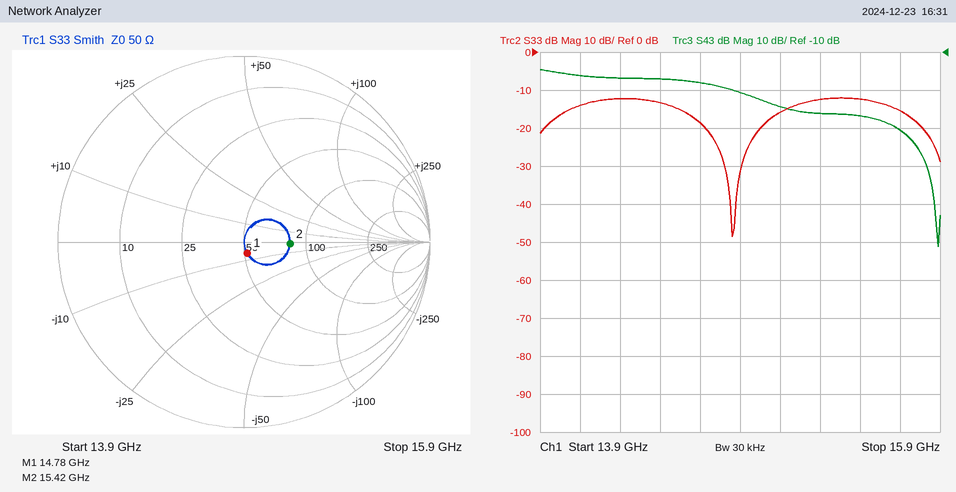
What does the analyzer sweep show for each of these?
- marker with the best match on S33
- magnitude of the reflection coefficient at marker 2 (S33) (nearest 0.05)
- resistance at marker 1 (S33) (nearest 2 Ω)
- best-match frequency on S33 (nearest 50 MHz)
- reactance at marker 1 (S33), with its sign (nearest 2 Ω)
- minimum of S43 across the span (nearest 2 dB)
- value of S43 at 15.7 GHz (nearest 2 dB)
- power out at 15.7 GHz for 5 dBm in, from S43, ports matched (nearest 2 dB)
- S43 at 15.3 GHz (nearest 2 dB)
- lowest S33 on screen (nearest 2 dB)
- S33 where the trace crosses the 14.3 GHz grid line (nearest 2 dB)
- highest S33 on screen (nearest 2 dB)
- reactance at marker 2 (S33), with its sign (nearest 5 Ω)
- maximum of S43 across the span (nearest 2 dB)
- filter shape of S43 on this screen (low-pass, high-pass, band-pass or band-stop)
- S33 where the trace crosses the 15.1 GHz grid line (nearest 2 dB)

marker 1
0.25
52 Ω
14.85 GHz
-6 Ω
-62 dB
-30 dB
-26 dBm
-26 dB
-48 dB
-12 dB
-12 dB
0 Ω
-14 dB
low-pass
-16 dB
